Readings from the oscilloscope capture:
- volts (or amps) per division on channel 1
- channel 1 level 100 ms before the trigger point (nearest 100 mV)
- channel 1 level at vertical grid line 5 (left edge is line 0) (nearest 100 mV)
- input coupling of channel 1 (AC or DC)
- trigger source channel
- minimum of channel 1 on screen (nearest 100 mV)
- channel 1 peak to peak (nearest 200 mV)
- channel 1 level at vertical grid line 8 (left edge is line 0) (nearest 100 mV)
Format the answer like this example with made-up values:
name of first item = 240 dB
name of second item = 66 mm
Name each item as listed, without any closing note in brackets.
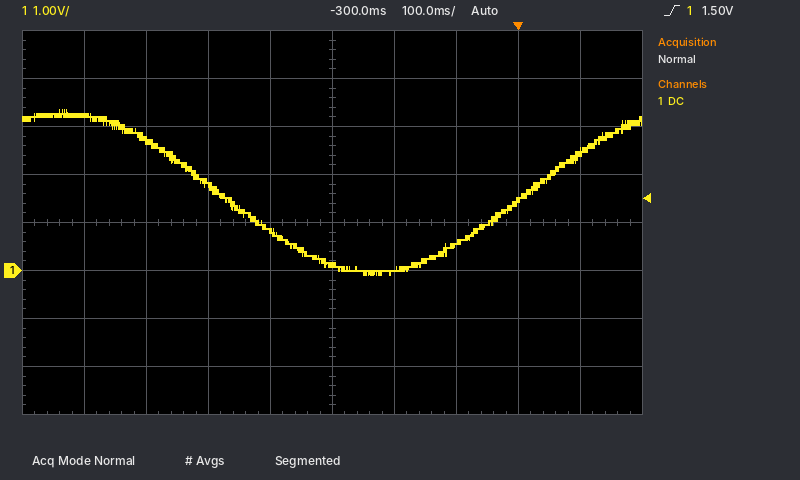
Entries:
volts (or amps) per division on channel 1 = 1 V
channel 1 level 100 ms before the trigger point = 600 mV
channel 1 level at vertical grid line 5 (left edge is line 0) = 100 mV
input coupling of channel 1 = DC
trigger source channel = channel 1
minimum of channel 1 on screen = -100 mV
channel 1 peak to peak = 3.4 V
channel 1 level at vertical grid line 8 (left edge is line 0) = 1.4 V
